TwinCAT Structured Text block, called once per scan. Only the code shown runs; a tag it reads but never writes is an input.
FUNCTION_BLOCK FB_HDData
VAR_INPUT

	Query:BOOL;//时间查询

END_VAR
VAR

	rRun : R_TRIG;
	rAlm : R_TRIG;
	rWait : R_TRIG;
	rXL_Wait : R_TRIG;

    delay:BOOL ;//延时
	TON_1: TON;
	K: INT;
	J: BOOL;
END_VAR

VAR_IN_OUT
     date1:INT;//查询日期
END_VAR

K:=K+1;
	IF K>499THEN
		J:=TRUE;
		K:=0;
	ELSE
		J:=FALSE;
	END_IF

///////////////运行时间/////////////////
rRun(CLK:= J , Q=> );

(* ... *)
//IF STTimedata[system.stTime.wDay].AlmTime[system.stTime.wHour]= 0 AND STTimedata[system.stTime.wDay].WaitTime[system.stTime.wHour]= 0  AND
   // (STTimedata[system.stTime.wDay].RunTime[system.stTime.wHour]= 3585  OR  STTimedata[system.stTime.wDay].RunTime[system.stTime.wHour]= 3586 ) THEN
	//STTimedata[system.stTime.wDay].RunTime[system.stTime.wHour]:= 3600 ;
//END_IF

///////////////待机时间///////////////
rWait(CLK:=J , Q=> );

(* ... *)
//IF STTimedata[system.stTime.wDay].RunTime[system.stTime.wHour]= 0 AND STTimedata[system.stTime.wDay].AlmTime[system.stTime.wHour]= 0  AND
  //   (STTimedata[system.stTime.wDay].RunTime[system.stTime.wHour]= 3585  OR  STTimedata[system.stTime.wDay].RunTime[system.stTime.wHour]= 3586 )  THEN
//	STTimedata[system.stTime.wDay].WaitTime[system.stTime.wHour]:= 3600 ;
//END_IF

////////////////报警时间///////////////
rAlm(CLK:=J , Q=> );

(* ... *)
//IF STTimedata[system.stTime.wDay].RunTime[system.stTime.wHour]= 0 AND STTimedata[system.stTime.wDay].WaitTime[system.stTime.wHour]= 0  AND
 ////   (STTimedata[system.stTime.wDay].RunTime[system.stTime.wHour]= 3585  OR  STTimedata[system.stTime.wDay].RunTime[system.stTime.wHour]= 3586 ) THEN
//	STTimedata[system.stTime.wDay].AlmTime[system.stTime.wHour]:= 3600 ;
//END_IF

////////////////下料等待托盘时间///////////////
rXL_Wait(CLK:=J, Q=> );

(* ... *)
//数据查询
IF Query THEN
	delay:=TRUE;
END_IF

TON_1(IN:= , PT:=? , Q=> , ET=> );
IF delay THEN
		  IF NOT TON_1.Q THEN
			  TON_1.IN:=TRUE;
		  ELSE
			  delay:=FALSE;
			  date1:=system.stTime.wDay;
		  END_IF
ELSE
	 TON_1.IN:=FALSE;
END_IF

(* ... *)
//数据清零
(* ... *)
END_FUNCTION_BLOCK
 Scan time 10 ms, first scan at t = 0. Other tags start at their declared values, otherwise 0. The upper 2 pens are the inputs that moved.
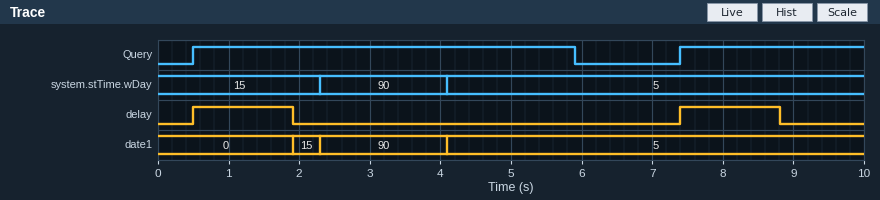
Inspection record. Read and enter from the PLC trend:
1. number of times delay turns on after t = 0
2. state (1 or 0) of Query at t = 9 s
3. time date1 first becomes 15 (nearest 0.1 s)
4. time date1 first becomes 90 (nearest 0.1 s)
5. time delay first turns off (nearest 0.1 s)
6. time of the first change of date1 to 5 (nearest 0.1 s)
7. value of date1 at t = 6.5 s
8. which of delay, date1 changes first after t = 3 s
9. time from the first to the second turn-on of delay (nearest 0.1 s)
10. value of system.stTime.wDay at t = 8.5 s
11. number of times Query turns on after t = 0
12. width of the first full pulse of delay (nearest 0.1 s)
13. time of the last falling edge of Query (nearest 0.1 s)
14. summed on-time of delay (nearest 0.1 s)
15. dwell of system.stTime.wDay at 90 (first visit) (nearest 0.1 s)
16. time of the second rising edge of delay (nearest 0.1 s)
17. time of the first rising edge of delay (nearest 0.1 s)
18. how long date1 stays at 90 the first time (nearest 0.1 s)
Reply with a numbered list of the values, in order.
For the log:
1. 2
2. 1
3. 1.9 s
4. 2.3 s
5. 1.9 s
6. 4.1 s
7. 5
8. date1
9. 6.9 s
10. 5
11. 2
12. 1.4 s
13. 5.9 s
14. 2.8 s
15. 1.8 s
16. 7.4 s
17. 0.5 s
18. 1.8 s
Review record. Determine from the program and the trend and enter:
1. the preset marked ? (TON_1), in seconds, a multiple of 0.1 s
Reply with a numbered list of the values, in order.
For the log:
1. 1.4 s
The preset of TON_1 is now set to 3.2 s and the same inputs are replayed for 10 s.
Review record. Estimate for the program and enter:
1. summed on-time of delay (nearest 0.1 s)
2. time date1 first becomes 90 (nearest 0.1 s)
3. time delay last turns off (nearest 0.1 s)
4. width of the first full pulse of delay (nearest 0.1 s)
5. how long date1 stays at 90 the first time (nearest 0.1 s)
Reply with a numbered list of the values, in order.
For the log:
1. 5.8 s
2. 3.7 s
3. 3.7 s
4. 3.2 s
5. 0.4 s
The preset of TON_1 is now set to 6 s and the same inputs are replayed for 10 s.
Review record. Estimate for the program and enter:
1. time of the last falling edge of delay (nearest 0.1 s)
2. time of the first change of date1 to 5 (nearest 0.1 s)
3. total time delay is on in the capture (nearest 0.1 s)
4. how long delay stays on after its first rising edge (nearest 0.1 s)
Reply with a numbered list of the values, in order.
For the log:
1. 6.5 s
2. 6.5 s
3. 8.6 s
4. 6.0 s
